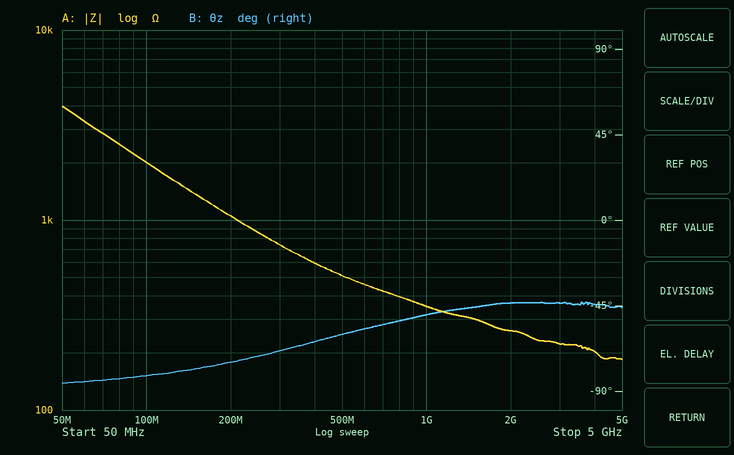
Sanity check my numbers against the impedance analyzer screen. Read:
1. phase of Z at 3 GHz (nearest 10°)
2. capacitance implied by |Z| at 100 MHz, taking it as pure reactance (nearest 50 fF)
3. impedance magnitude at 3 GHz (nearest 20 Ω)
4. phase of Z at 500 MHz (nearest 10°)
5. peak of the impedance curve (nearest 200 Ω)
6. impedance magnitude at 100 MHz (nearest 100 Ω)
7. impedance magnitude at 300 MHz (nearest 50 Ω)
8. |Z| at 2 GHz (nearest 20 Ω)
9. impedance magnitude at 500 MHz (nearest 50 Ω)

-40°
800 fF
220 Ω
-60°
4.0 kΩ
2.0 kΩ
750 Ω
260 Ω
500 Ω
